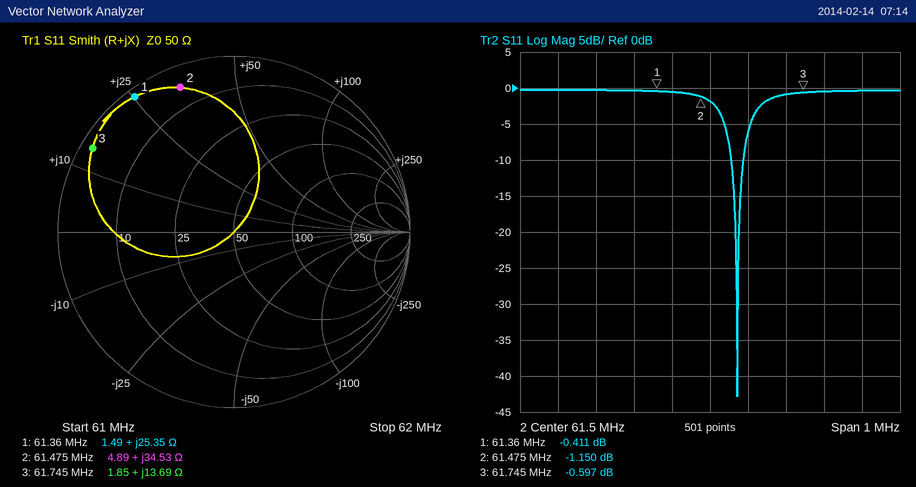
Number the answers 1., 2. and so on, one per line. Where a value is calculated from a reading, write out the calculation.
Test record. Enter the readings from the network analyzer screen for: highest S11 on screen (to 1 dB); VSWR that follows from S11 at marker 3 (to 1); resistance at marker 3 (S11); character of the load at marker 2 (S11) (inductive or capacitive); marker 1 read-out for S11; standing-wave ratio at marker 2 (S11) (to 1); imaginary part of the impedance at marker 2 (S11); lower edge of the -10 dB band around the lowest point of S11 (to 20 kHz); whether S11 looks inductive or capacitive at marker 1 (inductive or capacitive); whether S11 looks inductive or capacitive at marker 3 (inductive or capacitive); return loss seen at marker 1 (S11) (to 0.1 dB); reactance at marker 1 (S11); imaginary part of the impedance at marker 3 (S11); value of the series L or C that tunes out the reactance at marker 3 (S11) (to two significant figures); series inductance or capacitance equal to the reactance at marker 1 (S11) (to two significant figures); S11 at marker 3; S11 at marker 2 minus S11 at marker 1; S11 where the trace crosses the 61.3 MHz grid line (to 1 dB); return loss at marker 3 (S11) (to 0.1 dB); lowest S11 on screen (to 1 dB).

1. 0 dB
2. (1 + 0.9336)/(1 − 0.9336) ≈ 29
3. 1.85 Ω
4. inductive
5. -0.411 dB
6. 15
7. +34.53 Ω
8. 61.56 MHz
9. inductive
10. inductive
11. 0.4 dB
12. +25.35 Ω
13. +13.69 Ω
14. C = 1/(2π × 61.745 MHz × 13.69 Ω) ≈ 188 pF, so 190 pF to two significant figures
15. L = 25.35 Ω/(2π × 61.36 MHz) ≈ 66 nH
16. -0.597 dB
17. -1.15 − (-0.411) = -0.739 dB
18. 0 dB
19. 0.6 dB
20. -43 dB
